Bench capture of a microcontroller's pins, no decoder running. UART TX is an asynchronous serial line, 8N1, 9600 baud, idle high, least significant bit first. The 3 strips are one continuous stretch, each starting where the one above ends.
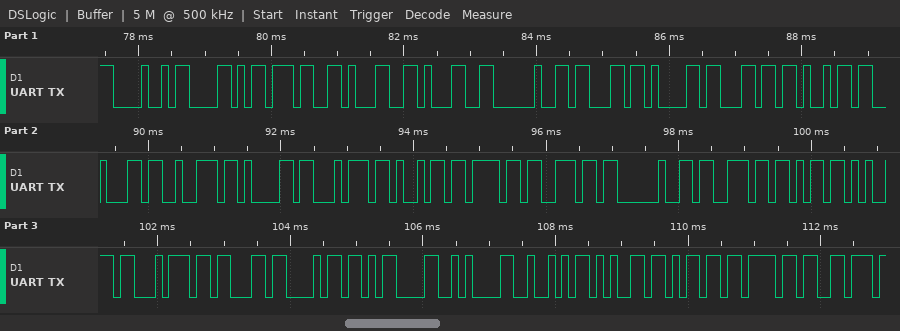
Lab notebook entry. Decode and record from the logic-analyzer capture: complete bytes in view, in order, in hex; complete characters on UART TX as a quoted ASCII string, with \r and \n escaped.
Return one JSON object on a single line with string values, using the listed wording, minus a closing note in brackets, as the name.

{"complete bytes in view, in order, in hex": "48 58 37 31 31 20 63 61 6C 69 62 72 61 74 69 6F 6E 20 73 6B 65 74 63 68 0D 0A 52 65 6D 6F 76", "complete characters on UART TX as a quoted ASCII string, with \\r and \\n escaped": "\"HX711 calibration sketch\\r\\nRemov\""}
